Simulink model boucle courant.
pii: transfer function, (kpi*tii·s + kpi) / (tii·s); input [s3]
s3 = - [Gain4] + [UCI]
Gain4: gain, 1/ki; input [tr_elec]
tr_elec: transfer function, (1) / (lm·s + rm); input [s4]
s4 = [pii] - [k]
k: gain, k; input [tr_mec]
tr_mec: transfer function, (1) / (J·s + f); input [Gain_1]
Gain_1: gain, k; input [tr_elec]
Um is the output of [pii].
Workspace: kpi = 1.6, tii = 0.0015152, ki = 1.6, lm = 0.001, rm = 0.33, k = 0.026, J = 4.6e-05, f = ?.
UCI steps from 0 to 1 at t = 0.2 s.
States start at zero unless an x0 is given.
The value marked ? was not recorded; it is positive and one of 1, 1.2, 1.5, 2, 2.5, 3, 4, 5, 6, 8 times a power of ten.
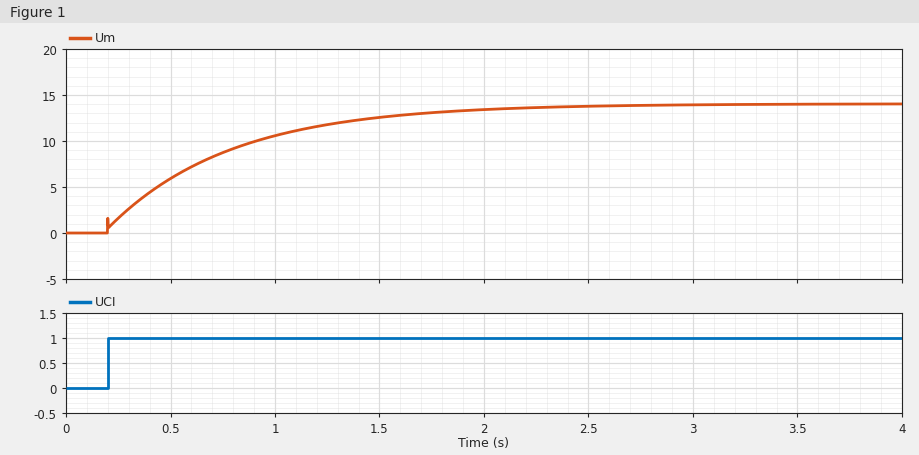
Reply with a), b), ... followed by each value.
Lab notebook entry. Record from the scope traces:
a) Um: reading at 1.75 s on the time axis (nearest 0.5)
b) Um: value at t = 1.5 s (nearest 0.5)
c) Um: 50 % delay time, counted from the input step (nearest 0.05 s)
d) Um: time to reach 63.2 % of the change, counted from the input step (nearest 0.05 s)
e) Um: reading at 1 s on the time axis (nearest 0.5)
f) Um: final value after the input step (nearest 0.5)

a) 13.0
b) 12.5
c) 0.40 s
d) 0.55 s
e) 10.5
f) 14.0
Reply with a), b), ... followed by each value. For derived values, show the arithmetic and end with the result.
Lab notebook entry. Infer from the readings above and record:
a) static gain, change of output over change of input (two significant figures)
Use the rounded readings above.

a) (14 - 0) / (1 - 0) = 14
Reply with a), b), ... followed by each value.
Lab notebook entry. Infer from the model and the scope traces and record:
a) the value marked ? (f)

a) 8e-05
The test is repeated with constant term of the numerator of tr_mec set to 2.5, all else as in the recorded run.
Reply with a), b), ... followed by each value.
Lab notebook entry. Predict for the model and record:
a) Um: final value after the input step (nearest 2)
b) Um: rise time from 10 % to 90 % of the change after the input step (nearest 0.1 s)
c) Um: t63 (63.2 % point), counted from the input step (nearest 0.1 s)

a) 34
b) 1.3 s
c) 0.6 s
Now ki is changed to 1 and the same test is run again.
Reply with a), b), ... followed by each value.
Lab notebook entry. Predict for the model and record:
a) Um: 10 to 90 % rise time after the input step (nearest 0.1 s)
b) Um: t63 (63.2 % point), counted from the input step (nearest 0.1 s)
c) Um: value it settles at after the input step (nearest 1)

a) 1.3 s
b) 0.6 s
c) 9
